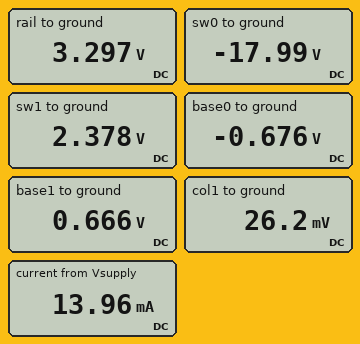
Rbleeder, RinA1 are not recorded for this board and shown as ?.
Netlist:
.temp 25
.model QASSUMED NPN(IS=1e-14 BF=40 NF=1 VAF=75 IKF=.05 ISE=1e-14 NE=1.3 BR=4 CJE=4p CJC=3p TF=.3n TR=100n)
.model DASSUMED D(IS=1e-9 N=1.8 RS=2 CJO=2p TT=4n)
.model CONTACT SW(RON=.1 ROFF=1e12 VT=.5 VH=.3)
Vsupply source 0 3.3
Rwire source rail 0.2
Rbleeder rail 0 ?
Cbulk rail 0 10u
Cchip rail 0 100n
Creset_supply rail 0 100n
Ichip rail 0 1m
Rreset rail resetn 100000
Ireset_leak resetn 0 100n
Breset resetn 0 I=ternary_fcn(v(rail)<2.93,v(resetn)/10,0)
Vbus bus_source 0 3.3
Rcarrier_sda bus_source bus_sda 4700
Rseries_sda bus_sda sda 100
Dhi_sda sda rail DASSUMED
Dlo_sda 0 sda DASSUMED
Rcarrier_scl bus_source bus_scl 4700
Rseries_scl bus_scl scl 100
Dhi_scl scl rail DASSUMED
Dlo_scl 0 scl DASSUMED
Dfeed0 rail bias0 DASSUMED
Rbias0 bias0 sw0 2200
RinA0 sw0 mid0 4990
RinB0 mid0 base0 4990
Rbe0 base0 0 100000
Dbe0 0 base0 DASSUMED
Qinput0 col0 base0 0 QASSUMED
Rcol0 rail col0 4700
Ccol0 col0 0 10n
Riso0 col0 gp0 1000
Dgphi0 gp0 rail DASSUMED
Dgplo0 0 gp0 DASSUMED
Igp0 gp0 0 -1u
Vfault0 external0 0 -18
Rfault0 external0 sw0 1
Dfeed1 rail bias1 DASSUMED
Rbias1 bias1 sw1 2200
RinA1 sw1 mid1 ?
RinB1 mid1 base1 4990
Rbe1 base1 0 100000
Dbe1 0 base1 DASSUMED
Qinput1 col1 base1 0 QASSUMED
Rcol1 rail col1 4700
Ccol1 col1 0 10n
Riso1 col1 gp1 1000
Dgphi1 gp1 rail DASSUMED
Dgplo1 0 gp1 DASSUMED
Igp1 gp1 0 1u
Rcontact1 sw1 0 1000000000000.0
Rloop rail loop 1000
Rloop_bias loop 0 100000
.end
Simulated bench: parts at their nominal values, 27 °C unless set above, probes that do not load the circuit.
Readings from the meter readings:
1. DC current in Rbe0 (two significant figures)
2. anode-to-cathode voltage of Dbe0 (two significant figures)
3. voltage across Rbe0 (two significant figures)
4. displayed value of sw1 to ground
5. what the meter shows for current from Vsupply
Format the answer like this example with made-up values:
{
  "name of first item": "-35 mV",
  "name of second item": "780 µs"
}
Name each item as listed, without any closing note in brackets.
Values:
{
  "DC current in Rbe0": "6.8 µA",
  "anode-to-cathode voltage of Dbe0": "680 mV",
  "voltage across Rbe0": "680 mV",
  "displayed value of sw1 to ground": "2.378 V",
  "what the meter shows for current from Vsupply": "13.96 mA"
}
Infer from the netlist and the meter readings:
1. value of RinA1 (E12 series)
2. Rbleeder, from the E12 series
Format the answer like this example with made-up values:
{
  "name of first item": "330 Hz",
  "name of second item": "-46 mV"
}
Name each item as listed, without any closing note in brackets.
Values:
{
  "value of RinA1": "5.6 kΩ",
  "Rbleeder, from the E12 series": "1.2 kΩ"
}
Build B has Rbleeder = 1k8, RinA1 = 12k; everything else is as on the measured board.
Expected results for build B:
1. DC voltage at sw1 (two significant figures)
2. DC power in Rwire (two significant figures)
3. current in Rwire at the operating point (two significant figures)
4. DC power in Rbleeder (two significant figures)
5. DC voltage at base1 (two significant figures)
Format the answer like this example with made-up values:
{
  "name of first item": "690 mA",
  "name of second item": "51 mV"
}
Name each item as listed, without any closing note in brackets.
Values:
{
  "DC voltage at sw1": "2.5 V",
  "DC power in Rwire": "34 µW",
  "current in Rwire at the operating point": "13 mA",
  "DC power in Rbleeder": "6.0 mW",
  "DC voltage at base1": "660 mV"
}
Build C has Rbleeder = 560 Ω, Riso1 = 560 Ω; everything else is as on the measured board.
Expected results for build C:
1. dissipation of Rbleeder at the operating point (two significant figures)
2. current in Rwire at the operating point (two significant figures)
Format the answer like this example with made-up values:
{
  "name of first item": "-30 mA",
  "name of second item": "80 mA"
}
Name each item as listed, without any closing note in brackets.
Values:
{
  "dissipation of Rbleeder at the operating point": "19 mW",
  "current in Rwire at the operating point": "17 mA"
}
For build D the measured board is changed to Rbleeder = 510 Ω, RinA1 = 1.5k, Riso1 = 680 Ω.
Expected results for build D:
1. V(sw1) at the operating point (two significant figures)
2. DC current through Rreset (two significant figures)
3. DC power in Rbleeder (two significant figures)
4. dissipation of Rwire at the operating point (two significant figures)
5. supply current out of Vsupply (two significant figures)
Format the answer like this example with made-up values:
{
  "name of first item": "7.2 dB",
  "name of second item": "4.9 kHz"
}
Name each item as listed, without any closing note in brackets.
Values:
{
  "V(sw1) at the operating point": "2.2 V",
  "DC current through Rreset": "100 nA",
  "DC power in Rbleeder": "21 mW",
  "dissipation of Rwire at the operating point": "63 µW",
  "supply current out of Vsupply": "18 mA"
}
